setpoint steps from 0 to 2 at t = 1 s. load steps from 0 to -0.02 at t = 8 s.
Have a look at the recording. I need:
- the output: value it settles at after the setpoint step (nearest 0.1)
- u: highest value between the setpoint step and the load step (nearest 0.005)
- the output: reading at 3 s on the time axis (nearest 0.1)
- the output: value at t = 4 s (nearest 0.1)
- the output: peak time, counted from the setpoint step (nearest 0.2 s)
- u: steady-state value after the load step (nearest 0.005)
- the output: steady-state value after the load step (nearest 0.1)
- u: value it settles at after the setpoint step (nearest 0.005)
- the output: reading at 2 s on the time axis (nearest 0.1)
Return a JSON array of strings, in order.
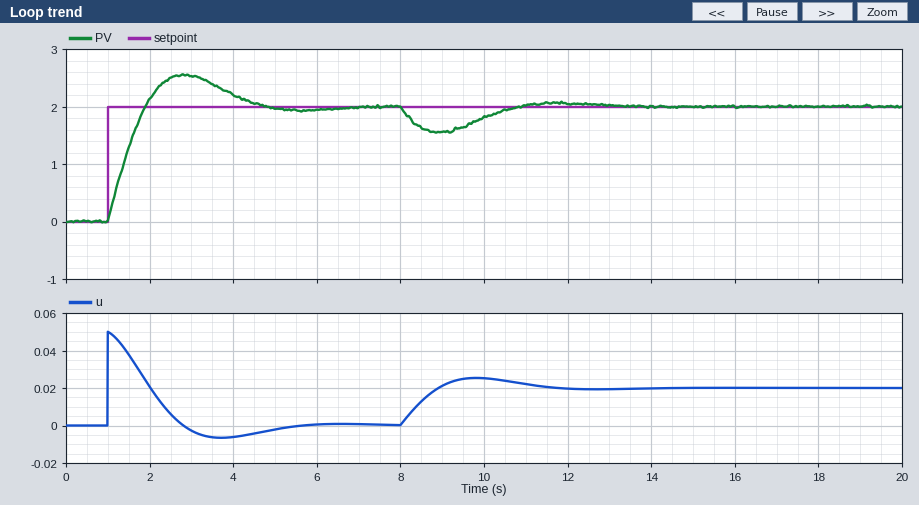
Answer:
["2.0", "0.050", "2.5", "2.2", "1.8 s", "0.020", "2.0", "0.000", "2.1"]
